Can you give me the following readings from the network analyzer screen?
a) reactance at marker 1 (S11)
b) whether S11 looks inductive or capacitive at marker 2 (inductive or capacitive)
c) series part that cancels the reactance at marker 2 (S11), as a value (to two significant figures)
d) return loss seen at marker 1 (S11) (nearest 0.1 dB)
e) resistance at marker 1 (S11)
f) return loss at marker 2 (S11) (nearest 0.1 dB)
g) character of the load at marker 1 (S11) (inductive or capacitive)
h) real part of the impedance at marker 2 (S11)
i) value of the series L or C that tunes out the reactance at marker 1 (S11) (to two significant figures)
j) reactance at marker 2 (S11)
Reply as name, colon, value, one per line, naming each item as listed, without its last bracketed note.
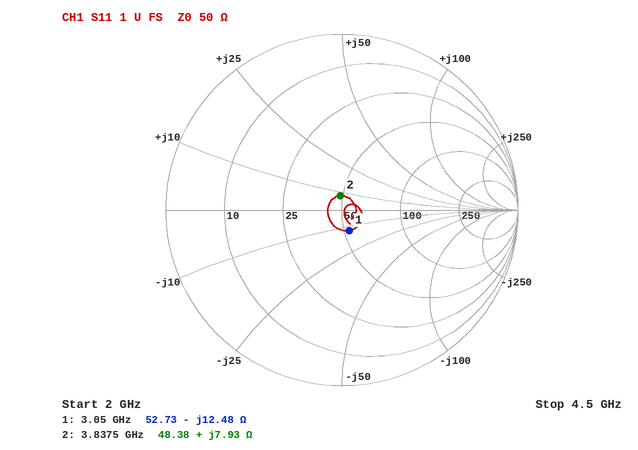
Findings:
reactance at marker 1: -12.48 Ω
whether S11 looks inductive or capacitive at marker 2: inductive
series part that cancels the reactance at marker 2 (S11), as a value: 5.2 pF
return loss seen at marker 1 (S11): 18.2 dB
resistance at marker 1: 52.73 Ω
return loss at marker 2 (S11): 21.7 dB
character of the load at marker 1 (S11): capacitive
real part of the impedance at marker 2: 48.38 Ω
value of the series L or C that tunes out the reactance at marker 1 (S11): 650 pH
reactance at marker 2: +7.93 Ω
